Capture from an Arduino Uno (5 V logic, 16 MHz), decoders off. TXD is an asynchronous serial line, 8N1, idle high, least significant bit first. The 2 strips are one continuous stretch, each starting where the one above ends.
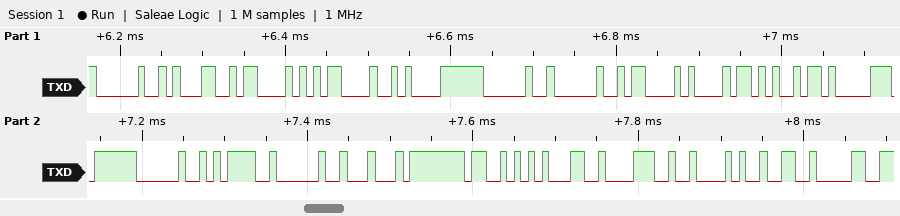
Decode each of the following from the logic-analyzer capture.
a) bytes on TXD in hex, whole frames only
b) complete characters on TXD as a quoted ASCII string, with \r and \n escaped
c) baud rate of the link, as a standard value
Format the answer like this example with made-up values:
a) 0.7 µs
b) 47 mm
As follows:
a) 20 31 43 0D 0A 20 20 43 68 69 70 20 3D 20 44 53 31 38 42 32 30
b) " 1C\r\n  Chip = DS18B20"
c) 115200 baud
